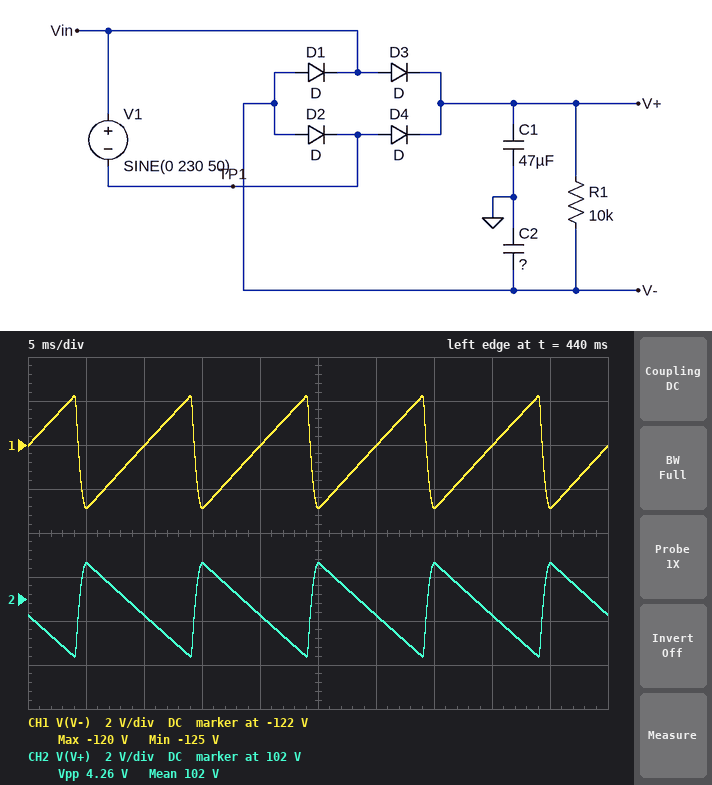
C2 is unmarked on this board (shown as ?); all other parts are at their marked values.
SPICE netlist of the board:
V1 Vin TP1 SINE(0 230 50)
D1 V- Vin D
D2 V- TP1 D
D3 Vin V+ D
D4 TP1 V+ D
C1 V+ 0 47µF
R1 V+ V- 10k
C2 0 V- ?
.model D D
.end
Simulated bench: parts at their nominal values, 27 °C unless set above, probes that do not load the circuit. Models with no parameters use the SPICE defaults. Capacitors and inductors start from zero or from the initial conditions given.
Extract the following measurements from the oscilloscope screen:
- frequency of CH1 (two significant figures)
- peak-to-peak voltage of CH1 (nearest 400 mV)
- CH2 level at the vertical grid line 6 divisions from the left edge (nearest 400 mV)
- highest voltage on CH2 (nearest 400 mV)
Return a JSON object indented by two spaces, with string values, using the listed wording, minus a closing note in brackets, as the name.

{
  "frequency of CH1": "100 Hz",
  "peak-to-peak voltage of CH1": "5.2 V",
  "CH2 level at the vertical grid line 6 divisions from the left edge": "101.2 V",
  "highest voltage on CH2": "103.6 V"
}
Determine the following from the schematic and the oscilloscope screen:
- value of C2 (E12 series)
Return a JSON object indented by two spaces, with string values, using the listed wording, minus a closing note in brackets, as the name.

{
  "value of C2": "39 µF"
}
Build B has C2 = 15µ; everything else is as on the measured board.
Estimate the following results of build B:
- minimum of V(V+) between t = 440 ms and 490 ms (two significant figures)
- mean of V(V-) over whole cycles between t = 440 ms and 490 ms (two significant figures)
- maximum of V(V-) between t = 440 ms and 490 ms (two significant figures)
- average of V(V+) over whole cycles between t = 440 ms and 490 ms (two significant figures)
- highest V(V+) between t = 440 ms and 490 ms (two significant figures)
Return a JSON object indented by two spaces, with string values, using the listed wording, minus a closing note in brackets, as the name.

{
  "minimum of V(V+) between t = 440 ms and 490 ms": "51 V",
  "mean of V(V-) over whole cycles between t = 440 ms and 490 ms": "-170 V",
  "maximum of V(V-) between t = 440 ms and 490 ms": "-160 V",
  "average of V(V+) over whole cycles between t = 440 ms and 490 ms": "53 V",
  "highest V(V+) between t = 440 ms and 490 ms": "55 V"
}
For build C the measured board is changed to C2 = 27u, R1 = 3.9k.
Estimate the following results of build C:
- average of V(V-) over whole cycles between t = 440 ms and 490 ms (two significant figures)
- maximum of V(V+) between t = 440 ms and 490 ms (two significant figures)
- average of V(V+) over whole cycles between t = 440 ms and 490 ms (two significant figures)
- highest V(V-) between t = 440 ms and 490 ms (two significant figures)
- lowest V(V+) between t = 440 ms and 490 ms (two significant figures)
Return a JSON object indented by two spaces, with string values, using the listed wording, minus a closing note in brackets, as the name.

{
  "average of V(V-) over whole cycles between t = 440 ms and 490 ms": "-140 V",
  "maximum of V(V+) between t = 440 ms and 490 ms": "83 V",
  "average of V(V+) over whole cycles between t = 440 ms and 490 ms": "79 V",
  "highest V(V-) between t = 440 ms and 490 ms": "-130 V",
  "lowest V(V+) between t = 440 ms and 490 ms": "74 V"
}
